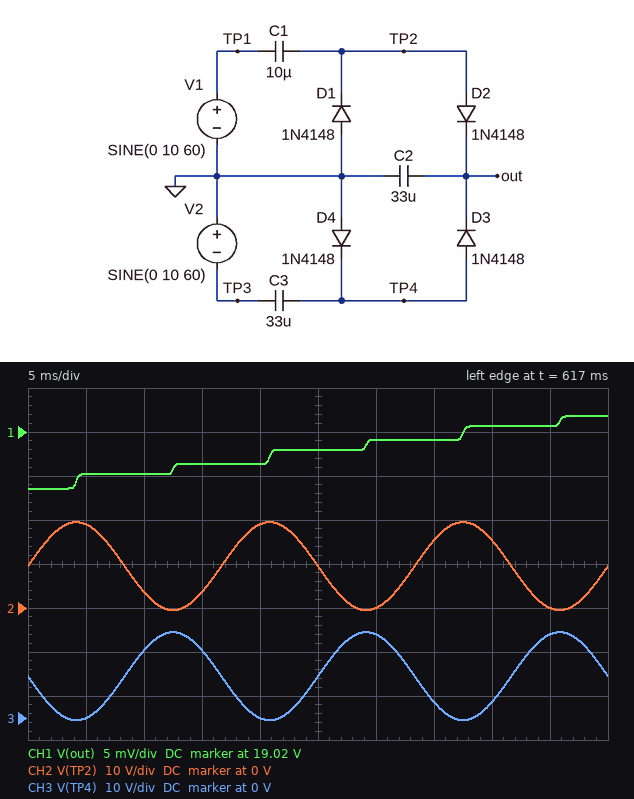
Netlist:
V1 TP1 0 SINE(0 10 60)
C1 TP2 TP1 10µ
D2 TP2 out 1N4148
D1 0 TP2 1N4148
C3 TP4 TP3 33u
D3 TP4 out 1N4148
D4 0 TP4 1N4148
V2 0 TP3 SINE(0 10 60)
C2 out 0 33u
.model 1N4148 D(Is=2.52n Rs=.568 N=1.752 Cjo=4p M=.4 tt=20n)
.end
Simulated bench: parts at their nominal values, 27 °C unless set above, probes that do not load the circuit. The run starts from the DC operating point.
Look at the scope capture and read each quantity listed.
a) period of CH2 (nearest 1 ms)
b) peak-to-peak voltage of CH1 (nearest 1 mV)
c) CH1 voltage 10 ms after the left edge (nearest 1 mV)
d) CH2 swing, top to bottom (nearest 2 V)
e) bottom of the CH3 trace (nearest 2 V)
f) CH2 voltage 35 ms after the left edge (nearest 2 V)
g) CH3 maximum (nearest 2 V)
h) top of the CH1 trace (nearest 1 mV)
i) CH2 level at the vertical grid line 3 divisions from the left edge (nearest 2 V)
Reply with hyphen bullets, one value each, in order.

- 17 ms
- 8 mV
- 19.015 V
- 20 V
- 0 V
- 16 V
- 20 V
- 19.022 V
- 4 V
